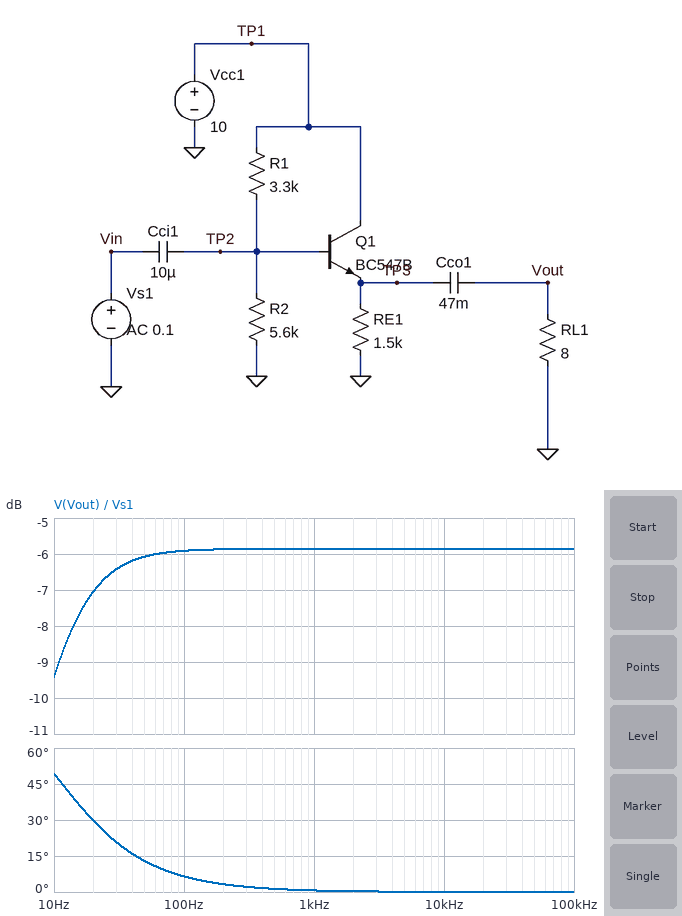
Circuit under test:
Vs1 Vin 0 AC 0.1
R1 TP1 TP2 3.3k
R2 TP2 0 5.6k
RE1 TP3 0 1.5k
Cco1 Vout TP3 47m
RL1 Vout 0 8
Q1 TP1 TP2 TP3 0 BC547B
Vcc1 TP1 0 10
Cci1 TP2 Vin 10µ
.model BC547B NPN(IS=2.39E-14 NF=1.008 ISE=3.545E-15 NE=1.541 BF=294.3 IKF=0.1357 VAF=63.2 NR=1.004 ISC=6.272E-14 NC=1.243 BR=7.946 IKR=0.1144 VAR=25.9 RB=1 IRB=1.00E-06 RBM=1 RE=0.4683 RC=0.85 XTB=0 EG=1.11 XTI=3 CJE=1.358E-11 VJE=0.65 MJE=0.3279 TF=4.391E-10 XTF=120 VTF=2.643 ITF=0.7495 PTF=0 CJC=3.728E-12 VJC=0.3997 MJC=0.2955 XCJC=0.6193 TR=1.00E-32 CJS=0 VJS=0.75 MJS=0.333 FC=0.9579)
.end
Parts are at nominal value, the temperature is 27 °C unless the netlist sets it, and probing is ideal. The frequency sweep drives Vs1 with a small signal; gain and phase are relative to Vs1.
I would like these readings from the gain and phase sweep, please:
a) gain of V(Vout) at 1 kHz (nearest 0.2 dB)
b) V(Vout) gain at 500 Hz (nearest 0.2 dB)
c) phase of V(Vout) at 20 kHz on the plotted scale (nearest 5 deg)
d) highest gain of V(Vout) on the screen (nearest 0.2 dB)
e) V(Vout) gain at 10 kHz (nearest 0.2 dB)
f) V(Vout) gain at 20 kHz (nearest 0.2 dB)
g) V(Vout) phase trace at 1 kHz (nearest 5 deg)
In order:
-5.8 dB
-5.8 dB
0 deg
-5.8 dB
-5.8 dB
-5.8 dB
0 deg
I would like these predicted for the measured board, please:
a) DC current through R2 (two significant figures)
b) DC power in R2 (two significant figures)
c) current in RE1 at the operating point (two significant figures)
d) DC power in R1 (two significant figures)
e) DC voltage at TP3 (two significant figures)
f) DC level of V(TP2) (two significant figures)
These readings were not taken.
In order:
1.1 mA
7.0 mW
3.7 mA
4.2 mW
5.6 V
6.3 V
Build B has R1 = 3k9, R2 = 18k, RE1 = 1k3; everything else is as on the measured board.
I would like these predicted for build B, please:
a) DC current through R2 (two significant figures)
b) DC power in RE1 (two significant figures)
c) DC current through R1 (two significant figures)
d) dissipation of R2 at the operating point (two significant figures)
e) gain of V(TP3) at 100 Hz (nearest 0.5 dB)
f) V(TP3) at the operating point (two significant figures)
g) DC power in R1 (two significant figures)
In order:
450 µA
43 mW
470 µA
3.7 mW
-4.5 dB
7.5 V
870 µW
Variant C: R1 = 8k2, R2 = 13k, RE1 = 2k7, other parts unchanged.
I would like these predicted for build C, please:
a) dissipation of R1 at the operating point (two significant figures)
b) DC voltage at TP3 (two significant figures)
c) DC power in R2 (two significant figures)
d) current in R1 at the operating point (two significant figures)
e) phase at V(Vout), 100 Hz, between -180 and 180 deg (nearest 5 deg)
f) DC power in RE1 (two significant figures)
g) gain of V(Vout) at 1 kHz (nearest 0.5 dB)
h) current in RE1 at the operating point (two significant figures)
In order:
1.9 mW
5.4 V
2.9 mW
480 µA
5 deg
11 mW
-8.5 dB
2.0 mA
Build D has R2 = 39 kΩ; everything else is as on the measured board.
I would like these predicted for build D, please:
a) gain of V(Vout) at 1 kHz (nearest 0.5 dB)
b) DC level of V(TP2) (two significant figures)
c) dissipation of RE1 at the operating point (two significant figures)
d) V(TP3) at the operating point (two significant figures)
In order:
-4.5 dB
9.2 V
48 mW
8.5 V
